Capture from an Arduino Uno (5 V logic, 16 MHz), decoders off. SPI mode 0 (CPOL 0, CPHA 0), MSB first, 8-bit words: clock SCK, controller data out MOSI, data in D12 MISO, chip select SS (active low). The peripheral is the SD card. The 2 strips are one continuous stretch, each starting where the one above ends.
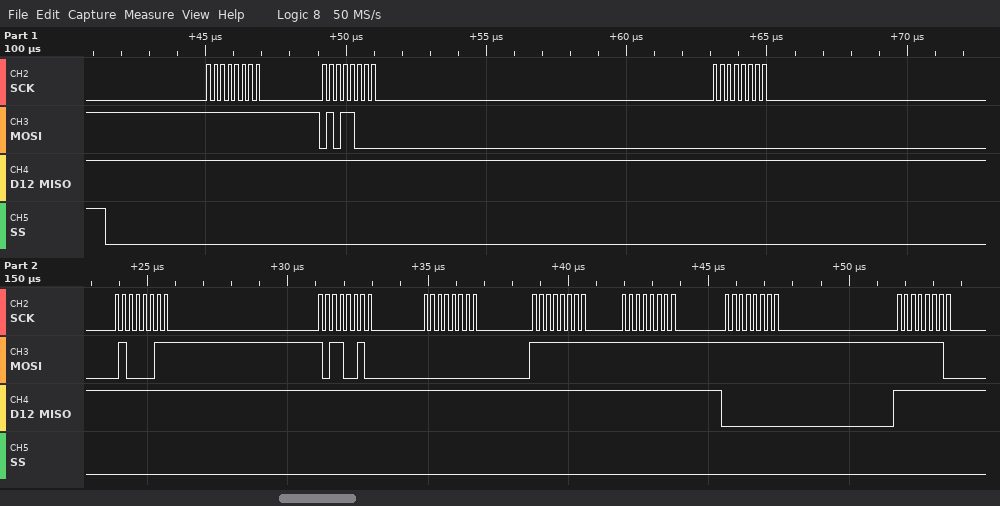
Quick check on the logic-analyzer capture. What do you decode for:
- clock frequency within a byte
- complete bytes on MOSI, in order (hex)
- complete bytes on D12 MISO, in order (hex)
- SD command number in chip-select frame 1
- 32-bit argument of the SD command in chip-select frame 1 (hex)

4 MHz
0xFF 0x58 0x00 0x43 0xB2 0x00 0xFF 0xFF 0xFF 0xFE
0xFF 0xFF 0xFF 0xFF 0xFF 0xFF 0xFF 0xFF 0x00 0xFF
CMD24
0x0043B200
